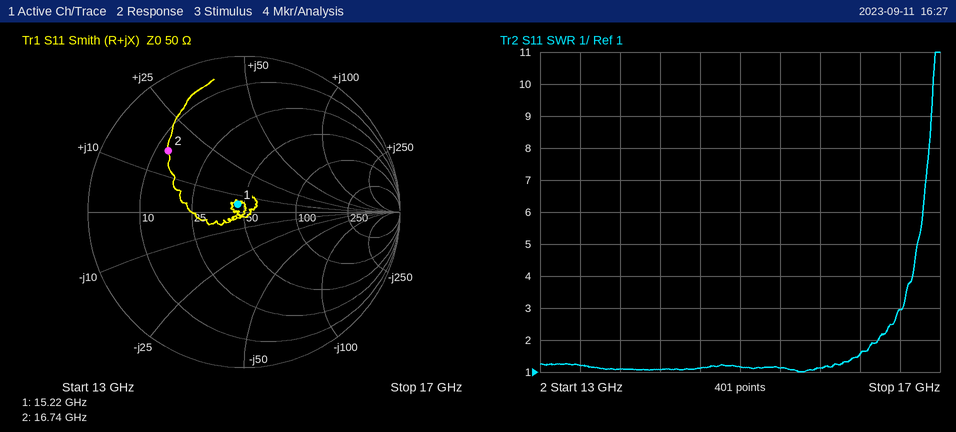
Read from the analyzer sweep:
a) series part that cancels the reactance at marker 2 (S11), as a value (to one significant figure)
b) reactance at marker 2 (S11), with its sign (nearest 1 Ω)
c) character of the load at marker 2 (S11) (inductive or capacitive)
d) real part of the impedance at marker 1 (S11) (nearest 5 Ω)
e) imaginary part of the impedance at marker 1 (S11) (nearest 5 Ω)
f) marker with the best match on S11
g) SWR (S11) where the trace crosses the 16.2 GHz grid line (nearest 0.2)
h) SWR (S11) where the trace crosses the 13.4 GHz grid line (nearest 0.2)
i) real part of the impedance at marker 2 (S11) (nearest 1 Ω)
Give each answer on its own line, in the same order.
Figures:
600 fF
+17 Ω
inductive
45 Ω
+5 Ω
marker 1
1.6
1.2
13 Ω
